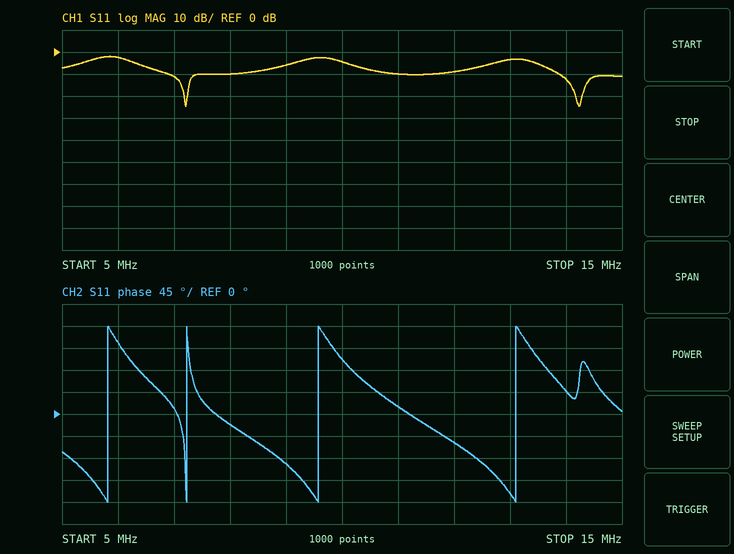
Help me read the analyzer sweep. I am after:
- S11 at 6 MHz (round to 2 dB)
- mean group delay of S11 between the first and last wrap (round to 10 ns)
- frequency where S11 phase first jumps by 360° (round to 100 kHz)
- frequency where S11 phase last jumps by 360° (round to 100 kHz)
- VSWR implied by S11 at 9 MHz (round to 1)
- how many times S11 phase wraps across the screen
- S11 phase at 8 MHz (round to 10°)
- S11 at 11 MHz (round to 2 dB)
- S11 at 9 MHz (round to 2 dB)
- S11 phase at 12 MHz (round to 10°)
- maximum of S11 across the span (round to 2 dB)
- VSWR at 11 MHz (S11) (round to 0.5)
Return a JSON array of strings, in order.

["-2 dB", "410 ns", "5.8 MHz", "13.1 MHz", "3", "4", "-20°", "-10 dB", "-6 dB", "-60°", "-2 dB", "2.0"]
